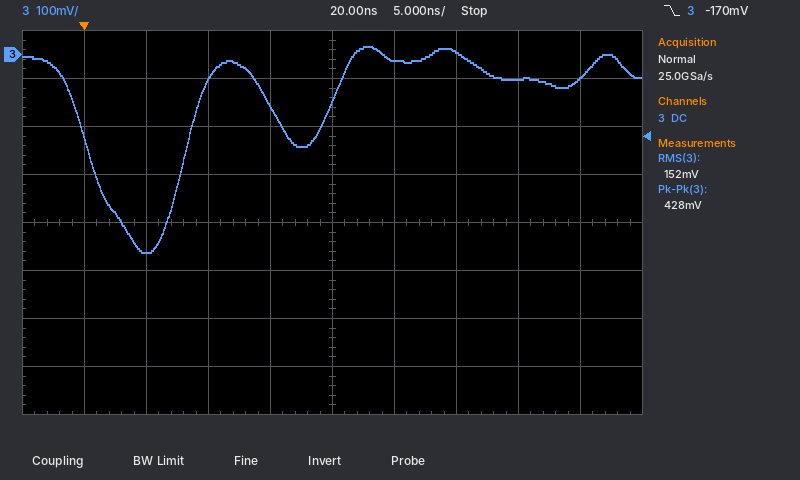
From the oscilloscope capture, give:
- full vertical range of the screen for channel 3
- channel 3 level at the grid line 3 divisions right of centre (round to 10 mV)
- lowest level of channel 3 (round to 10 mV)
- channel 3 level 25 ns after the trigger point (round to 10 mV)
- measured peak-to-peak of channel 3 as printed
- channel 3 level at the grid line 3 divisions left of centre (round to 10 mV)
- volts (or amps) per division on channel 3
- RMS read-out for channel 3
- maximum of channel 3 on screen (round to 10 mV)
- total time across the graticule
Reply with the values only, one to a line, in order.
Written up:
800 mV
-50 mV
-410 mV
-10 mV
428 mV
-410 mV
100 mV
152 mV
20 mV
50 ns
